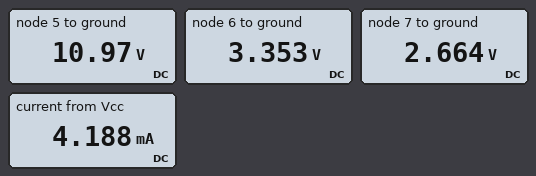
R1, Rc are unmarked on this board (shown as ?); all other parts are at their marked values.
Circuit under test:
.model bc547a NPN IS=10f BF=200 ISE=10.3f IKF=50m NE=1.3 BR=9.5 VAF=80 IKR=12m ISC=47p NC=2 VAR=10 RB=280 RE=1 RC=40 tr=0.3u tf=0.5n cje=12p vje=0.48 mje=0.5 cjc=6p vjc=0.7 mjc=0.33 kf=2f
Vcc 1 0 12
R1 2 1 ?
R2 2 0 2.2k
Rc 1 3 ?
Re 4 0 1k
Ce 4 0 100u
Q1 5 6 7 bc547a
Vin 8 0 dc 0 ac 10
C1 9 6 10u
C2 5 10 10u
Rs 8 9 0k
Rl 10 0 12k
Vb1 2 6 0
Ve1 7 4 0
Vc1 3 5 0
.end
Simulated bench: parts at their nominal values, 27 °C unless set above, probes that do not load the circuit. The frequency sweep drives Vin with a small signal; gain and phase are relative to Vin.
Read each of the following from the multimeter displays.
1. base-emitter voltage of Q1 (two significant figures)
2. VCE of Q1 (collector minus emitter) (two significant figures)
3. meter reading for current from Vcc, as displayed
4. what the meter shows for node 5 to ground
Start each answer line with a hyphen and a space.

- 690 mV
- 8.3 V
- 4.188 mA
- 10.97 V
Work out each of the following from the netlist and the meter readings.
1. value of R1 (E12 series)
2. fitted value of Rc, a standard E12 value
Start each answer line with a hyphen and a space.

- 5.6 kΩ
- 390 Ω
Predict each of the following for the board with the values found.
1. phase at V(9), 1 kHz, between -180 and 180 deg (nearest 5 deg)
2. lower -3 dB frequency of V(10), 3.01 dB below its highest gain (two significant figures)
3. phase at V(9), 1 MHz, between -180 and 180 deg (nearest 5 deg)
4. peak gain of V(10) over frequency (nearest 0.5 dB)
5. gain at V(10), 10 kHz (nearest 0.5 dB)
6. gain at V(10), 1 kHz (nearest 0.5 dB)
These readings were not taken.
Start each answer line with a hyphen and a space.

- 0 deg
- 130 Hz
- 0 deg
- 29.0 dB
- 29.0 dB
- 29.0 dB
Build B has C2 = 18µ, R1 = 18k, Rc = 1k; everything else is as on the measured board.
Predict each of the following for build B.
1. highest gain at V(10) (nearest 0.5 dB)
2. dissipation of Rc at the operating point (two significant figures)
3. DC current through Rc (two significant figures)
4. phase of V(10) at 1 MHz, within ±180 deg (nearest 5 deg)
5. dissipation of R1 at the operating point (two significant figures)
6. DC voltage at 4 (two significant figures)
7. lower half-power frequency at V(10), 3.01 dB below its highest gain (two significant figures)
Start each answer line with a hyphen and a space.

- 26.5 dB
- 420 µW
- 650 µA
- 170 deg
- 6.4 mW
- 650 mV
- 43 Hz
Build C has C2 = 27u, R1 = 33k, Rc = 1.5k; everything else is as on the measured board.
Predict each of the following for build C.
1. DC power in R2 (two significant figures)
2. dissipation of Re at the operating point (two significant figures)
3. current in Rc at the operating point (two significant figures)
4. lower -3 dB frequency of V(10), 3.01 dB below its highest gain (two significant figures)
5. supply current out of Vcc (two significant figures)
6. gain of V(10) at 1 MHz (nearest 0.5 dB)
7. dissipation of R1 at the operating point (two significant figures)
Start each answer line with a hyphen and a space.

- 250 µW
- 21 µW
- 140 µA
- 15 Hz
- 480 µA
- 17.0 dB
- 3.8 mW
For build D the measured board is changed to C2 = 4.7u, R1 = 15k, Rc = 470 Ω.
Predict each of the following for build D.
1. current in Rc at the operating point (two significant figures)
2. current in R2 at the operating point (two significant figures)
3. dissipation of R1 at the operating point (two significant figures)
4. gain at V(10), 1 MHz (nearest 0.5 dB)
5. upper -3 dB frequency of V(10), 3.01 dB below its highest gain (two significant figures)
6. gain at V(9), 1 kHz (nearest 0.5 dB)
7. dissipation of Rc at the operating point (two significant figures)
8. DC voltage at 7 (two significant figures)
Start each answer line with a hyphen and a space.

- 860 µA
- 690 µA
- 7.3 mW
- 22.5 dB
- 6.8 MHz
- 0 dB
- 350 µW
- 870 mV
